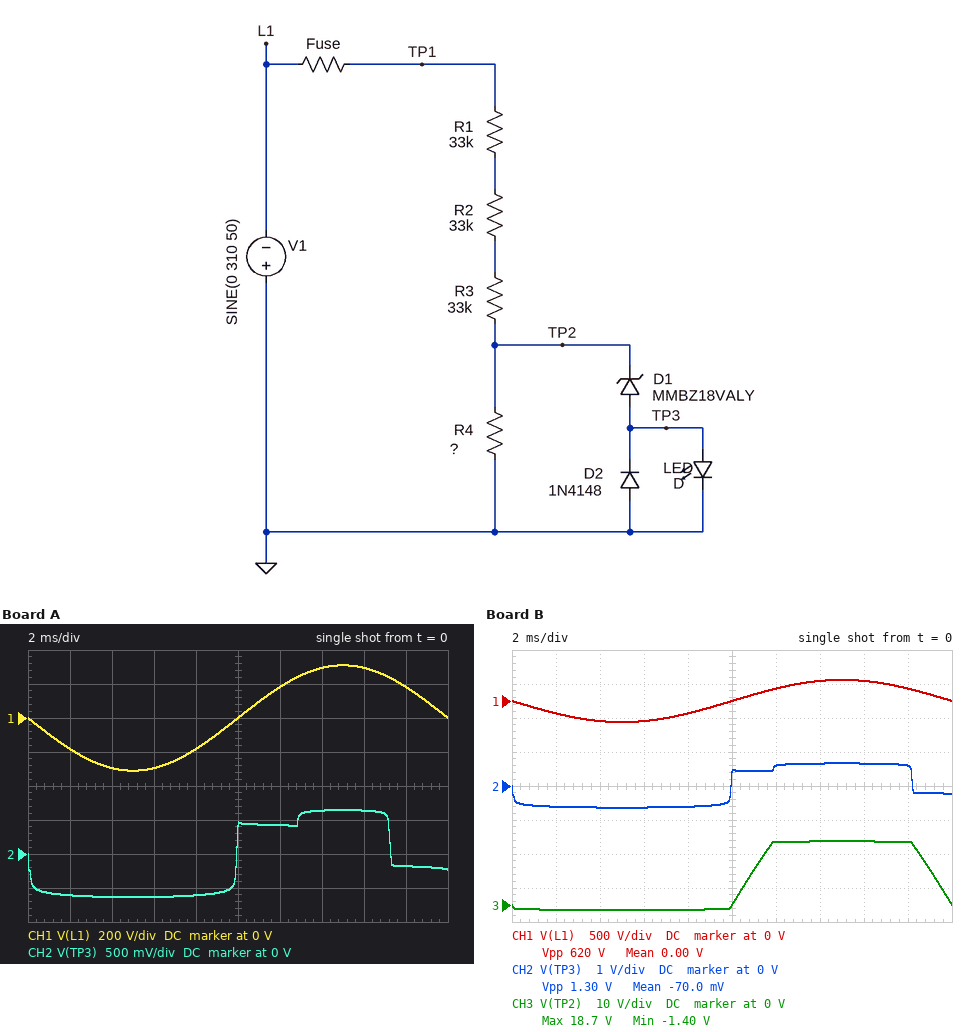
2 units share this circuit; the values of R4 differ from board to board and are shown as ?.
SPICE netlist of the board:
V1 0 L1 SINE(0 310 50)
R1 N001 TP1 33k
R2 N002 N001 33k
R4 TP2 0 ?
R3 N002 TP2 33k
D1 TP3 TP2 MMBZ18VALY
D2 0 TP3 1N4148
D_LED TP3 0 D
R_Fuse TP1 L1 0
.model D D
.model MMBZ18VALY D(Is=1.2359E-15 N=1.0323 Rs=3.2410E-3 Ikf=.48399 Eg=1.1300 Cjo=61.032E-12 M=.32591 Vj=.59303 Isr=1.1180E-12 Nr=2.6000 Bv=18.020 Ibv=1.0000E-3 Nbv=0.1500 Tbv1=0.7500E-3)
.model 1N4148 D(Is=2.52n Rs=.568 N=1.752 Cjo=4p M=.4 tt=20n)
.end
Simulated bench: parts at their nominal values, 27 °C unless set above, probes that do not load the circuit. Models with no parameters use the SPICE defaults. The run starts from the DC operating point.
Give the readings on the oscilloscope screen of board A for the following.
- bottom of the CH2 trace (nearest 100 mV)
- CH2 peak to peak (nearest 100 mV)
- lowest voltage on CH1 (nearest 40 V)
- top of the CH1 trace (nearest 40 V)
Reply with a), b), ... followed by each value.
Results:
a) -600 mV
b) 1.3 V
c) -320 V
d) 320 V
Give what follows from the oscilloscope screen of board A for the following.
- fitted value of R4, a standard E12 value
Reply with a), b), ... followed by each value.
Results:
a) 8.2 kΩ
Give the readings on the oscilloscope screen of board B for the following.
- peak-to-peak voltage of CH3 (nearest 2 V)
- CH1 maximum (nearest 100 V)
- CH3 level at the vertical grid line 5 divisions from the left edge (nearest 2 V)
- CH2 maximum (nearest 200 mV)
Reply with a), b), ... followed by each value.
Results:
a) 20 V
b) 300 V
c) 0 V
d) 600 mV
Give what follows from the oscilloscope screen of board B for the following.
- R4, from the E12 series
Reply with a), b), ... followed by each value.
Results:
a) 12 kΩ
